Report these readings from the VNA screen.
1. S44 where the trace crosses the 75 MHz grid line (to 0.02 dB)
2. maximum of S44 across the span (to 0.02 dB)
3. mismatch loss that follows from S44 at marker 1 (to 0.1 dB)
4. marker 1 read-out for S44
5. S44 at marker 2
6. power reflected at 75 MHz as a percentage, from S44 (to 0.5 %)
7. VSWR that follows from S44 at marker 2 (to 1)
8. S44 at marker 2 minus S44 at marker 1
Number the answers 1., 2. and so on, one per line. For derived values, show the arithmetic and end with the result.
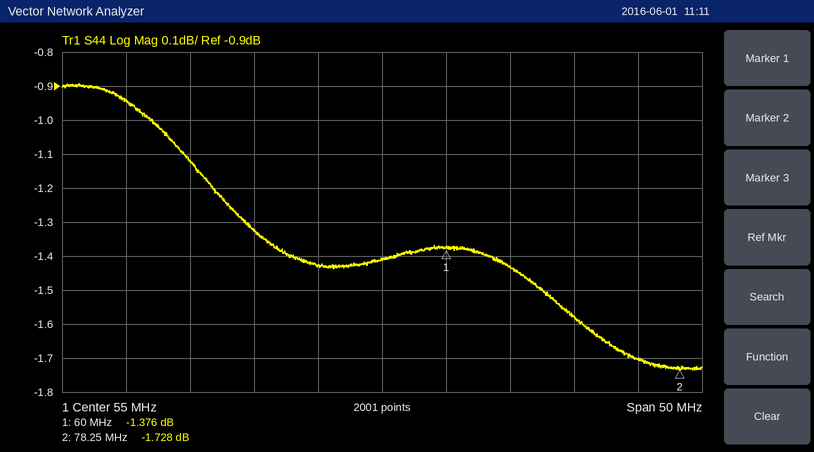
1. -1.70 dB
2. -0.90 dB
3. −10 log10(1 − 10^(-1.376/10)) ≈ 5.7 dB
4. -1.376 dB
5. -1.728 dB
6. 10^(-1.7/10) ≈ 67.6 %, so 67.5 % to the nearest 0.5 %
7. (1 + 0.8196)/(1 − 0.8196) ≈ 10
8. -1.728 − (-1.376) = -0.352 dB
